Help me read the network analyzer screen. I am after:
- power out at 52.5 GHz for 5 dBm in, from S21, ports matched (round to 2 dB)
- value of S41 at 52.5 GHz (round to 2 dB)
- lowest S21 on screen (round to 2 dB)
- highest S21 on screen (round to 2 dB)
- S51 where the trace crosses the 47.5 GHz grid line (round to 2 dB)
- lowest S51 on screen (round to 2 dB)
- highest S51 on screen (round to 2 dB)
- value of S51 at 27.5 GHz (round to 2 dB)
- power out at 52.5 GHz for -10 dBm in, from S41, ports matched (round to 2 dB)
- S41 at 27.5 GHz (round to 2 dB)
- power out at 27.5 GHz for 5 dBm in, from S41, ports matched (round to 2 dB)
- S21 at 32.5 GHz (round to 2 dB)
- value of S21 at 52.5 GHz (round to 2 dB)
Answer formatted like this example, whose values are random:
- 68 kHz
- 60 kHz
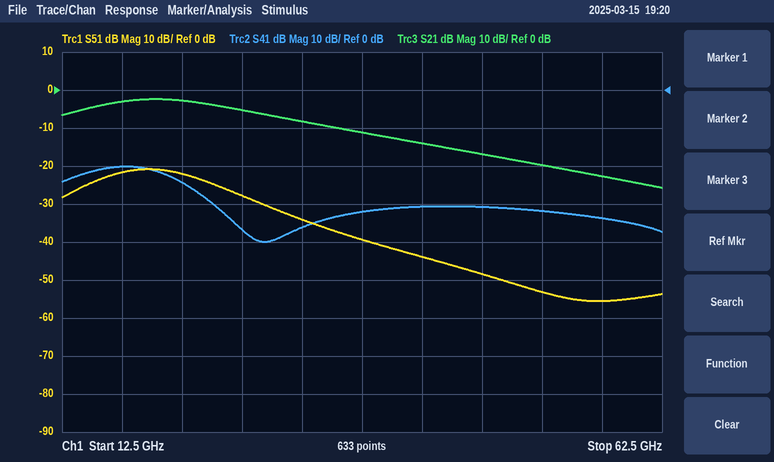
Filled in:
- -14 dBm
- -32 dB
- -26 dB
- -2 dB
- -48 dB
- -56 dB
- -20 dB
- -28 dB
- -42 dBm
- -36 dB
- -32 dBm
- -8 dB
- -20 dB
